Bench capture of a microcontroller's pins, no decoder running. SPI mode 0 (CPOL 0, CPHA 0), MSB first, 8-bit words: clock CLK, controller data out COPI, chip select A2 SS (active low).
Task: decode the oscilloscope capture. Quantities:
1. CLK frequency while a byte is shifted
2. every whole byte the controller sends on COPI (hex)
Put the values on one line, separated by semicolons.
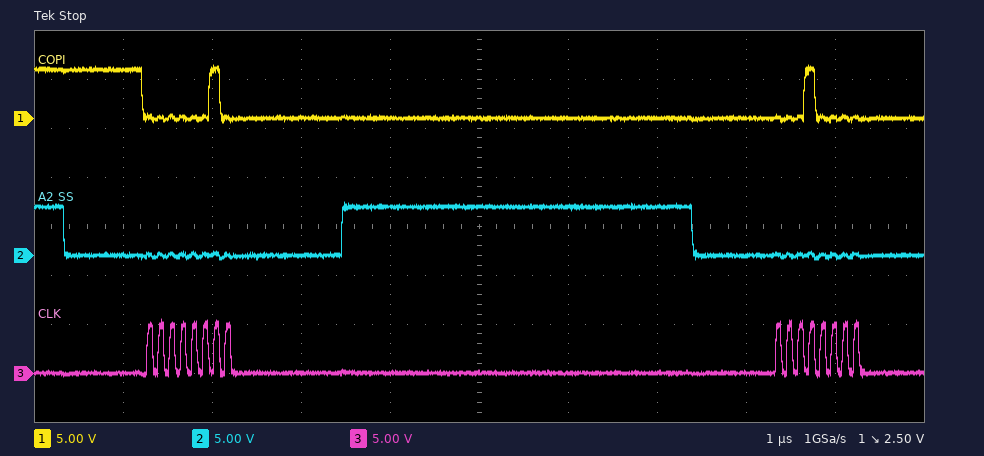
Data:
8 MHz; 02 10
